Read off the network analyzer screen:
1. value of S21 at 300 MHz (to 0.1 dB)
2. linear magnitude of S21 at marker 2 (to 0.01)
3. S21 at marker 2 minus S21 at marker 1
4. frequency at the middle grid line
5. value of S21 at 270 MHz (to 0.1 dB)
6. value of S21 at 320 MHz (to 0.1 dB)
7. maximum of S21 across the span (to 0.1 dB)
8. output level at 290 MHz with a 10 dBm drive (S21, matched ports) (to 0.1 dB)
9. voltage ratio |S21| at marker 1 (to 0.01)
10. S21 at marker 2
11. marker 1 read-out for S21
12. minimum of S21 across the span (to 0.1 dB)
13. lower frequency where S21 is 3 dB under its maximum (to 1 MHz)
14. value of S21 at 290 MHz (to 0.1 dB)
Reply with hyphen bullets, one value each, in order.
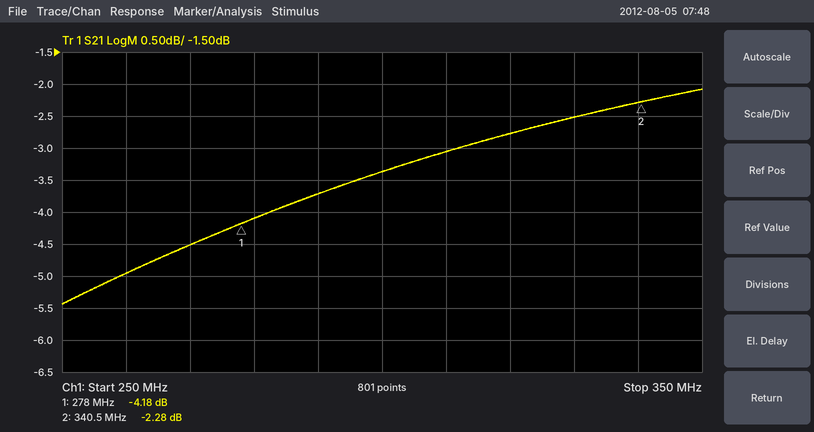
- -3.4 dB
- 0.77
- 1.90 dB
- 300 MHz
- -4.5 dB
- -2.8 dB
- -2.1 dB
- 6.3 dBm
- 0.62
- -2.28 dB
- -4.18 dB
- -5.4 dB
- 257 MHz
- -3.7 dB
